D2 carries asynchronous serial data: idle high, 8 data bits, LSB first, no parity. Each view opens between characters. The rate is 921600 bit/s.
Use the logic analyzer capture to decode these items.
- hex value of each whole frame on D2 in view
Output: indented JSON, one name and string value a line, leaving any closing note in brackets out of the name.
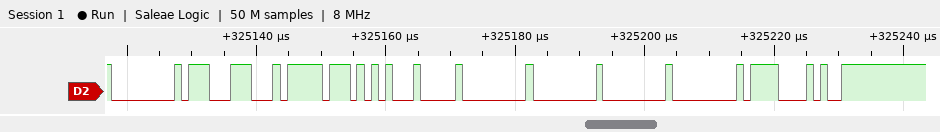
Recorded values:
{
  "hex value of each whole frame on D2 in view": "00, C7, F4, 57, 04, 00, 00, 00, 00, 0F, F9"
}
